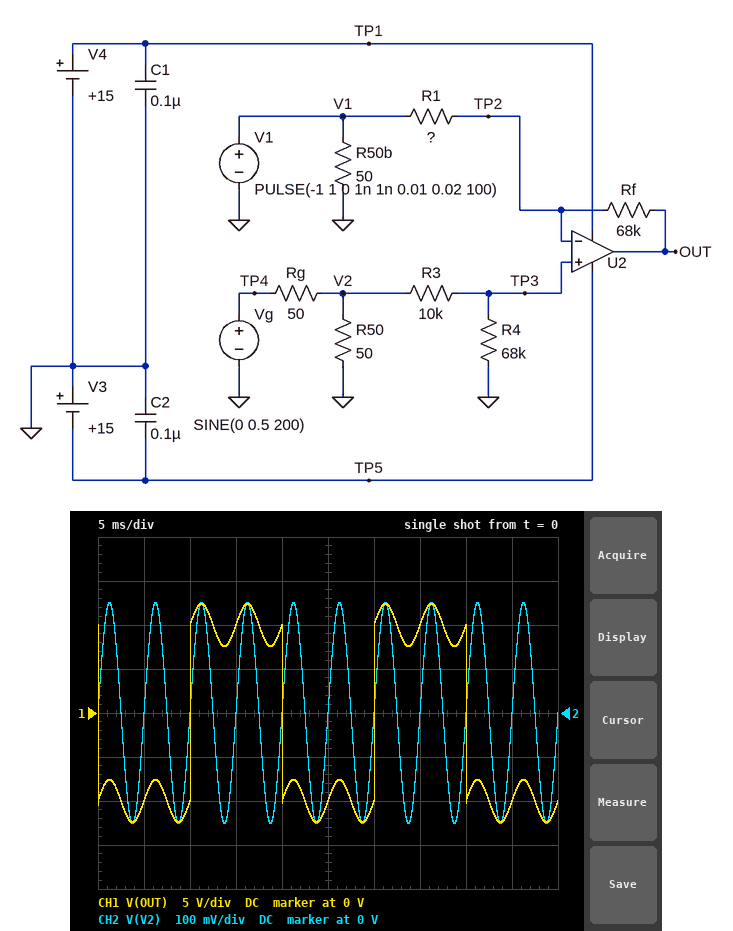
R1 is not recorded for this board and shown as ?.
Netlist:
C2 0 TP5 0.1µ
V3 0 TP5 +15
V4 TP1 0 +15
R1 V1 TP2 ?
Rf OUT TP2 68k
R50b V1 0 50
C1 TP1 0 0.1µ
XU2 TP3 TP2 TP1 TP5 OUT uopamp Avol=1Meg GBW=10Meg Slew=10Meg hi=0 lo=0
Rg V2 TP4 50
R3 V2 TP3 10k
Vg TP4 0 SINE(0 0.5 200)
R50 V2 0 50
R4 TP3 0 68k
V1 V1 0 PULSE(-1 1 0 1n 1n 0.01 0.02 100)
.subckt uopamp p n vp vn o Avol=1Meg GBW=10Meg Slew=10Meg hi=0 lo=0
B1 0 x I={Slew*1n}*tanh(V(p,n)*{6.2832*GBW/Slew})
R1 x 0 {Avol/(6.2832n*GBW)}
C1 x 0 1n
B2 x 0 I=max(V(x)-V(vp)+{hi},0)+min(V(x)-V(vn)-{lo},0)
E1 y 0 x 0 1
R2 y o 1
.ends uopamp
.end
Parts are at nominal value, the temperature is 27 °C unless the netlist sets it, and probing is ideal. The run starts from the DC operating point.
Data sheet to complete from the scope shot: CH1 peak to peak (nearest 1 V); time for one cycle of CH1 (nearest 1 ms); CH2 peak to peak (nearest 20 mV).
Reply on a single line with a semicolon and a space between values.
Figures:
25 V; 20 ms; 500 mV
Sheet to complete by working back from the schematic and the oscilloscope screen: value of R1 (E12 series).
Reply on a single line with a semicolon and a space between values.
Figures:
6.8 kΩ
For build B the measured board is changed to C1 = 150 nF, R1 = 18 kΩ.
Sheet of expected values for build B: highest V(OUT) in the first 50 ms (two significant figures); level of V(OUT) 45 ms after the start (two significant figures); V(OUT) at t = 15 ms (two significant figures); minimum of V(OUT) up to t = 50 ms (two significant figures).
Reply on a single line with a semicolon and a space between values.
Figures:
4.8 V; -3.8 V; 3.8 V; -4.8 V
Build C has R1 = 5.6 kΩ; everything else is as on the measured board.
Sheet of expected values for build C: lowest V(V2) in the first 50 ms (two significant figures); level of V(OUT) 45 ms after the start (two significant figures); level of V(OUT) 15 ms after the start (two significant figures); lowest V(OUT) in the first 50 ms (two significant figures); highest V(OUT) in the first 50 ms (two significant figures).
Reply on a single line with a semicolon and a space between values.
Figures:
-250 mV; -12 V; 12 V; -15 V; 15 V
